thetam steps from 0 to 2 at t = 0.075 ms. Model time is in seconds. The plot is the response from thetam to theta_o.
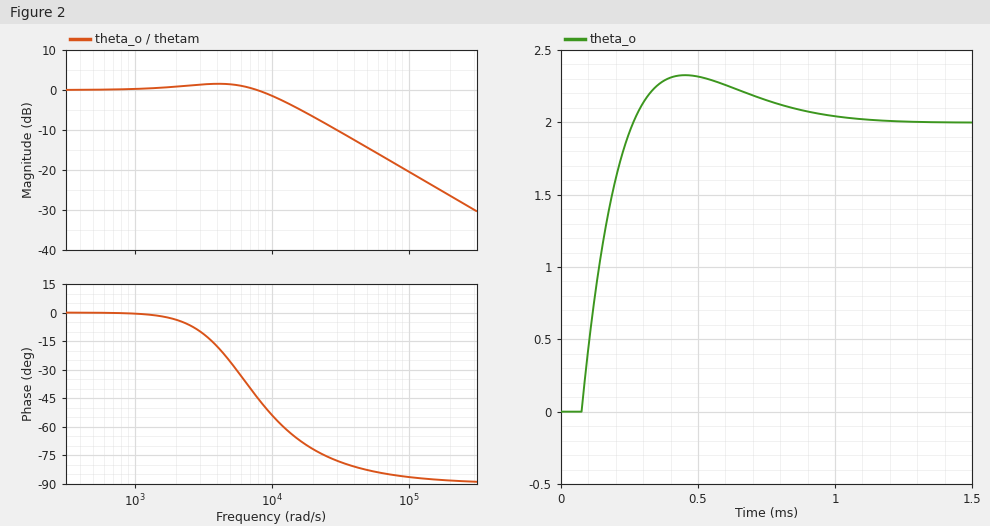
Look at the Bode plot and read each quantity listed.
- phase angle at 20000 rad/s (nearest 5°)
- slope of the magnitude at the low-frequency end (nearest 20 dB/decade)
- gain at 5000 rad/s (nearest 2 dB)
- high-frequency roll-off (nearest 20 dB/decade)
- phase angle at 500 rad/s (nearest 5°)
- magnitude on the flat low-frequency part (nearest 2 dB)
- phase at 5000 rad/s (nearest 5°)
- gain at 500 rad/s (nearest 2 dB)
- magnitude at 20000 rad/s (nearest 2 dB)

-70°
0 dB/decade
2 dB
-20 dB/decade
0°
0 dB
-25°
0 dB
-6 dB
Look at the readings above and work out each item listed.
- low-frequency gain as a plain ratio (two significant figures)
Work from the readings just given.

1.0
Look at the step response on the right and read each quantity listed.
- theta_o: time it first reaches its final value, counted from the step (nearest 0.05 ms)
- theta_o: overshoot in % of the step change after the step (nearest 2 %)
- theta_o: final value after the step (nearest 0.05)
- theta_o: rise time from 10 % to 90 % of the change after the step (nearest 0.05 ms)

0.20 ms
16 %
2.00
0.15 ms
